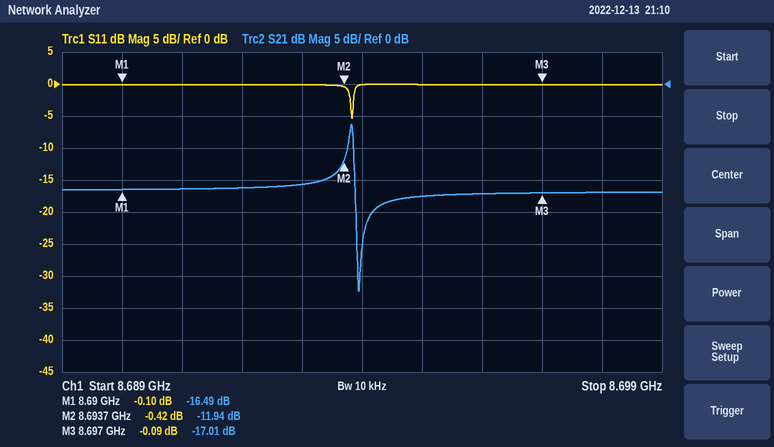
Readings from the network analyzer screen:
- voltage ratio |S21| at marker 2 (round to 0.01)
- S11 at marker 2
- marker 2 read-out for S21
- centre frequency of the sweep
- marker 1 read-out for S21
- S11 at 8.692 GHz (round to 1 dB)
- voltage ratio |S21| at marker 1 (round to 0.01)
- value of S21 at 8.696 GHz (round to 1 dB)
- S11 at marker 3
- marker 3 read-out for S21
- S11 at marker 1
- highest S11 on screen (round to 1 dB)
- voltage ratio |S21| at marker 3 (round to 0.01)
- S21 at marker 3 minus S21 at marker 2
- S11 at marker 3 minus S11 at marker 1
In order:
0.25
-0.42 dB
-11.94 dB
8.694 GHz
-16.49 dB
0 dB
0.15
-17 dB
-0.09 dB
-17.01 dB
-0.10 dB
0 dB
0.14
-5.07 dB
0.01 dB
